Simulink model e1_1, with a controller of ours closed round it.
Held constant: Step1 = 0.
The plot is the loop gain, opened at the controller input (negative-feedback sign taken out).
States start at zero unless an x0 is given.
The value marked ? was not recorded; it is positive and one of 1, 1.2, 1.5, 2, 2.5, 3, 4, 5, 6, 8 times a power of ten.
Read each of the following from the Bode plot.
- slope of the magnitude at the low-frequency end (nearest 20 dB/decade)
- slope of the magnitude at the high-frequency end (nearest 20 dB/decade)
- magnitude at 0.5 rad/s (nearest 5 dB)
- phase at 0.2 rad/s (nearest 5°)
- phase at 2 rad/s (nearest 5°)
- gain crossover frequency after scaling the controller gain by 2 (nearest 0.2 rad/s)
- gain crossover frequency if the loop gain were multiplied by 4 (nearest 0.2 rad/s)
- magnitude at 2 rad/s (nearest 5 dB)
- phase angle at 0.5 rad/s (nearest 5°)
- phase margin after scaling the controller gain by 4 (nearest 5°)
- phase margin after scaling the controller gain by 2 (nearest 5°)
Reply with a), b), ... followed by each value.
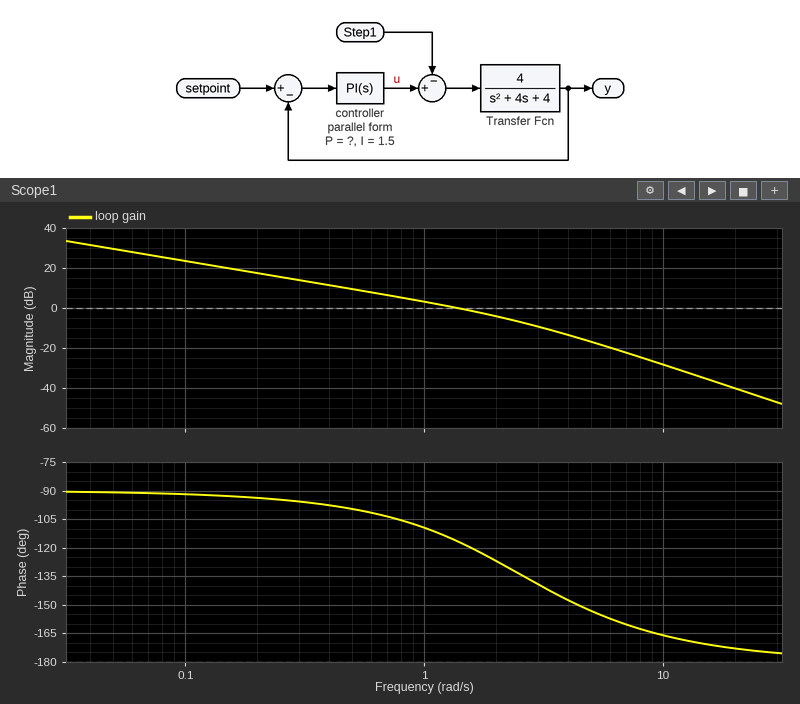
a) -20 dB/decade
b) -40 dB/decade
c) 10 dB
d) -95°
e) -125°
f) 2.4 rad/s
g) 3.6 rad/s
h) -5 dB
i) -100°
j) 35°
k) 50°
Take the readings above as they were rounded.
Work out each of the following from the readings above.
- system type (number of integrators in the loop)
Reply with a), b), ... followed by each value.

a) 1
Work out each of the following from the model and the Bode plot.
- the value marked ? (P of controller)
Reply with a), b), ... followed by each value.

a) 1
